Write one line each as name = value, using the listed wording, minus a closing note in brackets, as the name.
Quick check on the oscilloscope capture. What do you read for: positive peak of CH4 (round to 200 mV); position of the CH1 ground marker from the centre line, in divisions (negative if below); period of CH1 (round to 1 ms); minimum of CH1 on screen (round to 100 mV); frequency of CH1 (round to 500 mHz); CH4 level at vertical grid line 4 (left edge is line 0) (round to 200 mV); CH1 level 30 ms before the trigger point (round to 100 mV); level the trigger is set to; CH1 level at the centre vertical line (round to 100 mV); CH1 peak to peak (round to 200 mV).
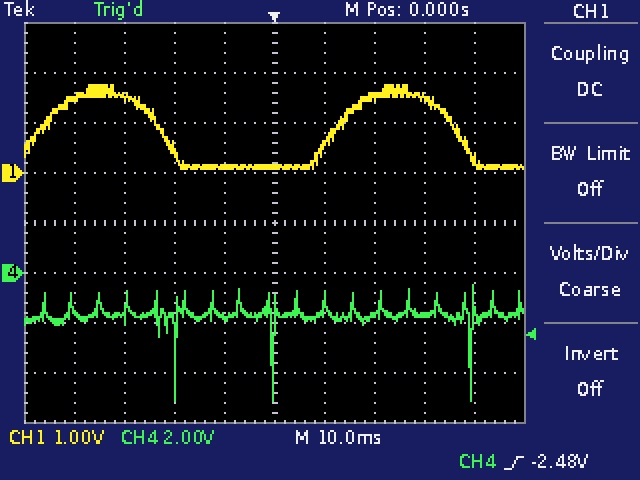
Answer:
positive peak of CH4 = -400 mV
position of the CH1 ground marker from the centre line, in divisions = +1.0 div
period of CH1 = 59 ms
minimum of CH1 on screen = 100 mV
frequency of CH1 = 17.0 Hz
CH4 level at vertical grid line 4 (left edge is line 0) = -1.8 V
CH1 level 30 ms before the trigger point = 1.5 V
level the trigger is set to = -2.48 V
CH1 level at the centre vertical line = 100 mV
CH1 peak to peak = 1.6 V
